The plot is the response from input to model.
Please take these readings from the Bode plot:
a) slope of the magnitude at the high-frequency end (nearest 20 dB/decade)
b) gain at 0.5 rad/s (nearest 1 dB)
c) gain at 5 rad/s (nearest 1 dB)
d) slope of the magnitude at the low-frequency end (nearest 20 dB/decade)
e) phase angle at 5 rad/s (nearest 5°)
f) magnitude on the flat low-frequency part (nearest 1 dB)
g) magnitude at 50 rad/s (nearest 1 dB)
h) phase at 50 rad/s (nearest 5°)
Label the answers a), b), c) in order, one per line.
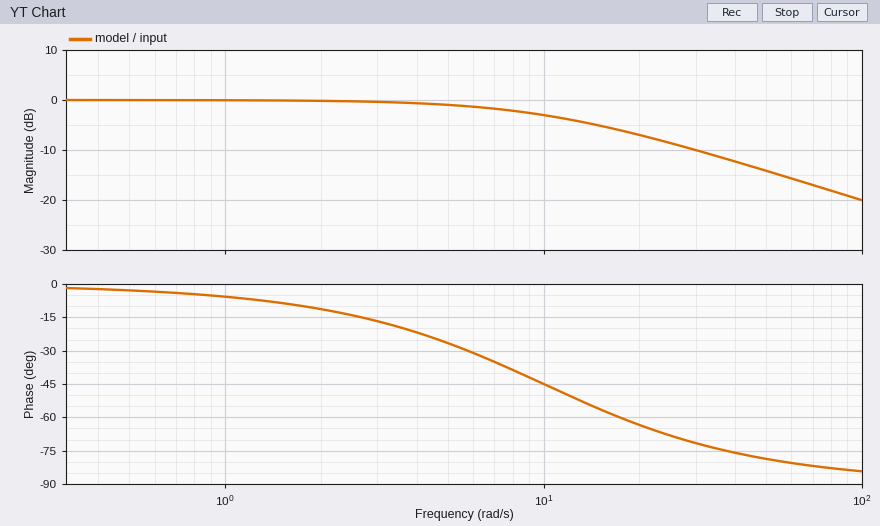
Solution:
a) -20 dB/decade
b) 0 dB
c) -1 dB
d) 0 dB/decade
e) -25°
f) 0 dB
g) -14 dB
h) -80°
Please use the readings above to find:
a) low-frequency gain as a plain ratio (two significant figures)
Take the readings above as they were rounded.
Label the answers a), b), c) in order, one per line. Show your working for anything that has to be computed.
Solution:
a) 10^(0 / 20) = 1.0
